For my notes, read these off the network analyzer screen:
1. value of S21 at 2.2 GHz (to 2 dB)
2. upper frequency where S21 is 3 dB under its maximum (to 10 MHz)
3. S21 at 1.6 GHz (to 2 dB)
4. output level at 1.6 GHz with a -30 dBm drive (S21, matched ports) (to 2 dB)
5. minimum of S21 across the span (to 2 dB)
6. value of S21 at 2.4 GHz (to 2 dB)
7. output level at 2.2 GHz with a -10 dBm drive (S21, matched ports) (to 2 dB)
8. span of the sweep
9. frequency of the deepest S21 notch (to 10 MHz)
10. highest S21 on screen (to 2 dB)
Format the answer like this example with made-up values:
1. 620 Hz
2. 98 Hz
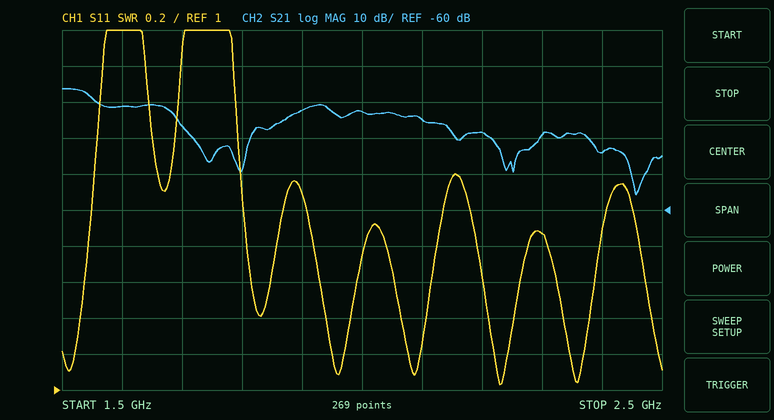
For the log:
1. -38 dB
2. 1.55 GHz
3. -32 dB
4. -62 dBm
5. -56 dB
6. -44 dB
7. -48 dBm
8. 1 GHz
9. 2.46 GHz
10. -26 dB
